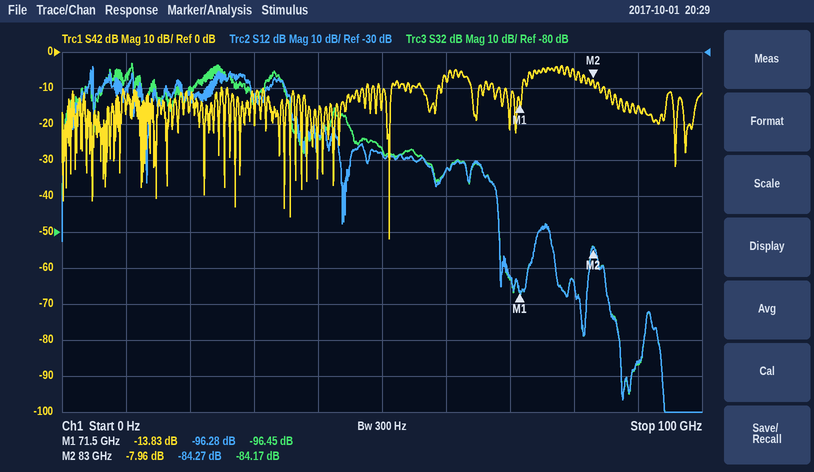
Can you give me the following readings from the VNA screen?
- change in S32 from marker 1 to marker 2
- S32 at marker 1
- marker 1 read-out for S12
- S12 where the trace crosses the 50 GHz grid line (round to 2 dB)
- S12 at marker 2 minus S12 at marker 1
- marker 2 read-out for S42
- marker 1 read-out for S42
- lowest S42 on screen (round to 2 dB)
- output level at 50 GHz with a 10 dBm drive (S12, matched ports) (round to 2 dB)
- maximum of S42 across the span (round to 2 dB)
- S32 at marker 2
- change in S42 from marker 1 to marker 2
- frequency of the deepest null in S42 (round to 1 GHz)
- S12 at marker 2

12.28 dB
-96.45 dB
-96.28 dB
-58 dB
12.01 dB
-7.96 dB
-13.83 dB
-52 dB
-48 dBm
-4 dB
-84.17 dB
5.87 dB
51 GHz
-84.27 dB
